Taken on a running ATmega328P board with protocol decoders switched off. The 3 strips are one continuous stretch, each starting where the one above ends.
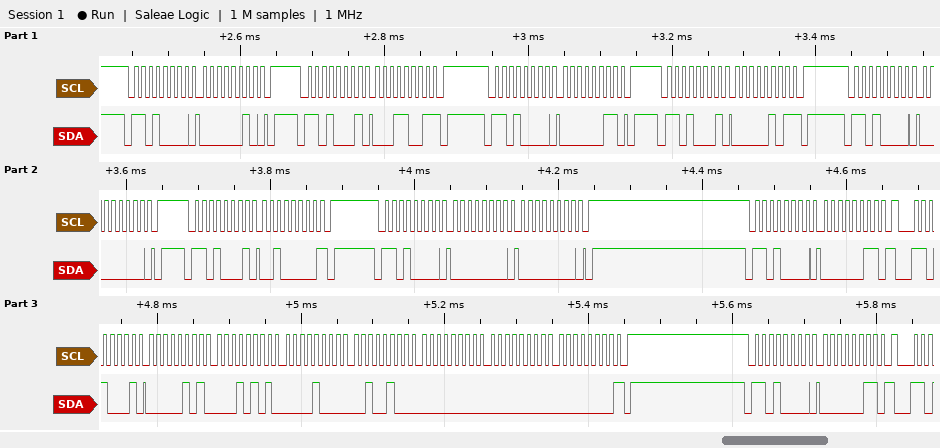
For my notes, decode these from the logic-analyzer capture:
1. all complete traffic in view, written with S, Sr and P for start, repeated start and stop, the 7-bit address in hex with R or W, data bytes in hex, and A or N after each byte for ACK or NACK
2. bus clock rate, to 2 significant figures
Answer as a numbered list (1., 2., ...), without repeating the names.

1. S 68W A 02 A P S 68R A 19 N P S 68W A 03 A P S 68R A 05 N P S 68W A 00 A P S 68R A 20 N P S 68W A 00 A 00 A P S 68W A 03 A Sr 68R A 05 A 15 A 08 A 24 A 00 A 00 A 00 N P S 68W A 03 A
2. 100 kHz
